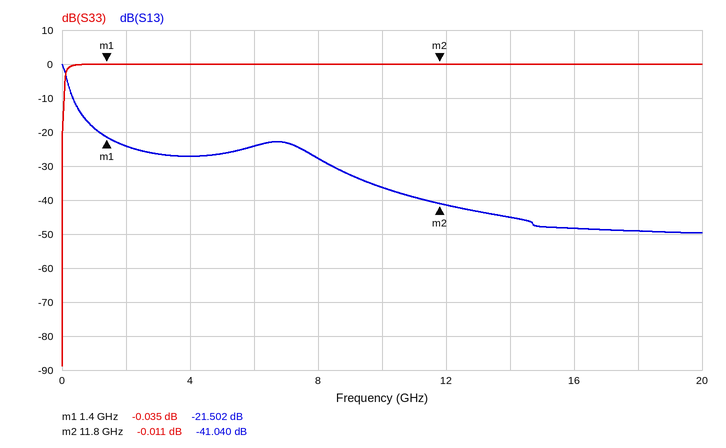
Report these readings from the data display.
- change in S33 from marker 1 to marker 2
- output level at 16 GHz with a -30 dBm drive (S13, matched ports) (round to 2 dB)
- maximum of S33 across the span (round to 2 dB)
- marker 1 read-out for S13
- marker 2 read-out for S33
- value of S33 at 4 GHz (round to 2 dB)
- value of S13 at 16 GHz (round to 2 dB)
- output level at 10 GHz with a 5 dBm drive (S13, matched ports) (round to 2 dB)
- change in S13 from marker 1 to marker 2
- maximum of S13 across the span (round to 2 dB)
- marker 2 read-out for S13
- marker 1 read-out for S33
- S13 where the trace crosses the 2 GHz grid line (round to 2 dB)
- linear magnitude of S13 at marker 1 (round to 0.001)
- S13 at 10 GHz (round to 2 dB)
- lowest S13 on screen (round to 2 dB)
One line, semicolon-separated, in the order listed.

0.024 dB; -78 dBm; 0 dB; -21.502 dB; -0.011 dB; 0 dB; -48 dB; -32 dBm; -19.538 dB; 0 dB; -41.040 dB; -0.035 dB; -24 dB; 0.084; -36 dB; -50 dB
